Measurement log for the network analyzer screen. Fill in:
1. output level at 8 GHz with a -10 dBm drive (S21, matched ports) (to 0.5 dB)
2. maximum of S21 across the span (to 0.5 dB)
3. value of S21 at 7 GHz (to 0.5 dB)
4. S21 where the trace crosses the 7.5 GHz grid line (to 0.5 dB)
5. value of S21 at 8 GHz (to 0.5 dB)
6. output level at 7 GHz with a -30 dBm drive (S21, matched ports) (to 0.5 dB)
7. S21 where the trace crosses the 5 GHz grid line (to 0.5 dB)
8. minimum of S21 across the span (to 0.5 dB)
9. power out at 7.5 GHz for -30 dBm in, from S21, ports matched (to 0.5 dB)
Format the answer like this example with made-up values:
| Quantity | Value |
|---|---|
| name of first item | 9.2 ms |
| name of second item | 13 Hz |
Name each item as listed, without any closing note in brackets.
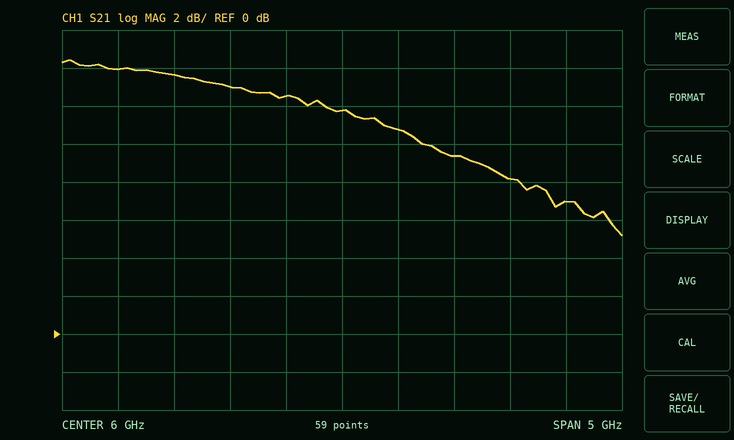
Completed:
| Quantity | Value |
|---|---|
| output level at 8 GHz with a -10 dBm drive (S21, matched ports) | -3.0 dBm |
| maximum of S21 across the span | 14.5 dB |
| value of S21 at 7 GHz | 9.5 dB |
| S21 where the trace crosses the 7.5 GHz grid line | 8.0 dB |
| value of S21 at 8 GHz | 7.0 dB |
| output level at 7 GHz with a -30 dBm drive (S21, matched ports) | -20.5 dBm |
| S21 where the trace crosses the 5 GHz grid line | 13.0 dB |
| minimum of S21 across the span | 5.0 dB |
| power out at 7.5 GHz for -30 dBm in, from S21, ports matched | -22.0 dBm |
